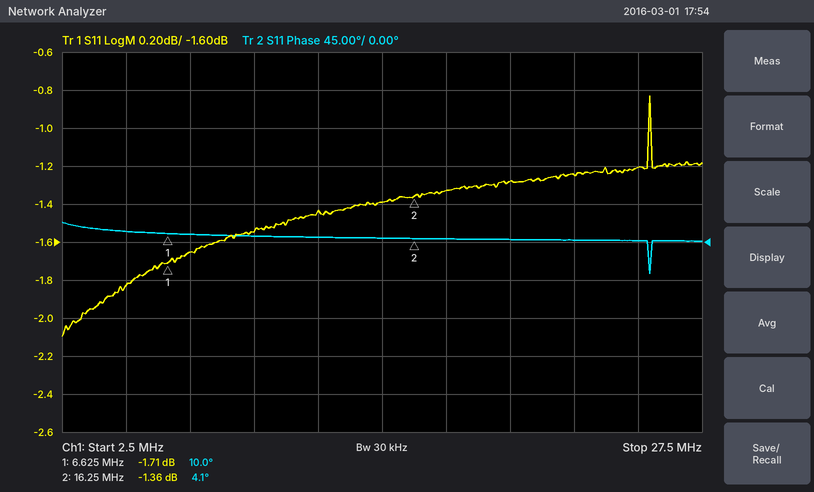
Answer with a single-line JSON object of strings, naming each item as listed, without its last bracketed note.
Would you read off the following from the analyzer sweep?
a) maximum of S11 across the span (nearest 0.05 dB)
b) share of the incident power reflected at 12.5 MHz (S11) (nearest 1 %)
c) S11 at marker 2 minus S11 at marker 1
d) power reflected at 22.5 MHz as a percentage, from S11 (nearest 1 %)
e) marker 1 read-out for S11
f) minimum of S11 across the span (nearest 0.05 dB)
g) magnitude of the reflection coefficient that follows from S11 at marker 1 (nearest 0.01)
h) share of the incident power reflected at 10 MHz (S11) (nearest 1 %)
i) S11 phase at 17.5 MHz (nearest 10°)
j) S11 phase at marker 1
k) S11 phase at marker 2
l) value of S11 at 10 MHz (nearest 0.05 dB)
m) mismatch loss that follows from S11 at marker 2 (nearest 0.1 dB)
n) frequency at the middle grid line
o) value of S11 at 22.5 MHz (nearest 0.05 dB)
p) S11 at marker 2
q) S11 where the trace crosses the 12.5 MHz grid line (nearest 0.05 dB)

{"maximum of S11 across the span": "-0.85 dB", "share of the incident power reflected at 12.5 MHz (S11)": "72 %", "S11 at marker 2 minus S11 at marker 1": "0.35 dB", "power reflected at 22.5 MHz as a percentage, from S11": "75 %", "marker 1 read-out for S11": "-1.71 dB", "minimum of S11 across the span": "-2.10 dB", "magnitude of the reflection coefficient that follows from S11 at marker 1": "0.82", "share of the incident power reflected at 10 MHz (S11)": "70 %", "S11 phase at 17.5 MHz": "0°", "S11 phase at marker 1": "10.0°", "S11 phase at marker 2": "4.1°", "value of S11 at 10 MHz": "-1.55 dB", "mismatch loss that follows from S11 at marker 2": "5.7 dB", "frequency at the middle grid line": "15 MHz", "value of S11 at 22.5 MHz": "-1.25 dB", "S11 at marker 2": "-1.36 dB", "S11 where the trace crosses the 12.5 MHz grid line": "-1.45 dB"}
